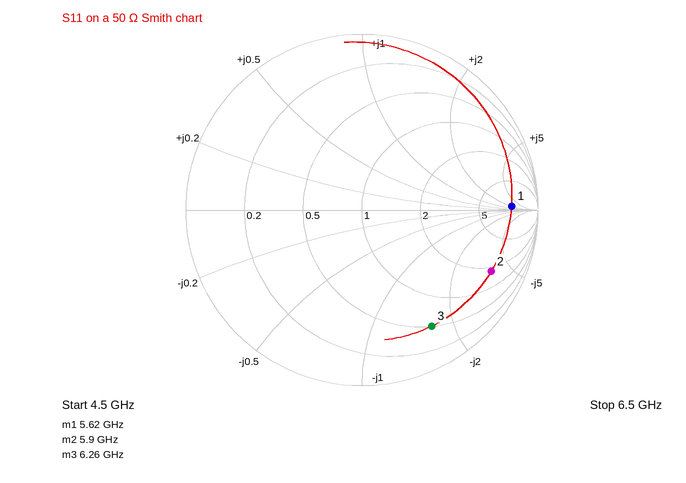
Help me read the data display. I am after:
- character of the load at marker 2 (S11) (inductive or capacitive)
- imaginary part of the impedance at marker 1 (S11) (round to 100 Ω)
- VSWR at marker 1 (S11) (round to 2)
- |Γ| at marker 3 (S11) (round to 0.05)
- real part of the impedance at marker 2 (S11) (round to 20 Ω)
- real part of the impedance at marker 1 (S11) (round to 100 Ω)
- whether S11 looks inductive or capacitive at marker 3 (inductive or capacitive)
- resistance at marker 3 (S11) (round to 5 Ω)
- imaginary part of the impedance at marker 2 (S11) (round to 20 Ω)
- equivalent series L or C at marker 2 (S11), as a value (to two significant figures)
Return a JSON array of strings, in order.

["capacitive", "+100 Ω", "12", "0.75", "80 Ω", "600 Ω", "capacitive", "25 Ω", "-180 Ω", "150 fF"]
